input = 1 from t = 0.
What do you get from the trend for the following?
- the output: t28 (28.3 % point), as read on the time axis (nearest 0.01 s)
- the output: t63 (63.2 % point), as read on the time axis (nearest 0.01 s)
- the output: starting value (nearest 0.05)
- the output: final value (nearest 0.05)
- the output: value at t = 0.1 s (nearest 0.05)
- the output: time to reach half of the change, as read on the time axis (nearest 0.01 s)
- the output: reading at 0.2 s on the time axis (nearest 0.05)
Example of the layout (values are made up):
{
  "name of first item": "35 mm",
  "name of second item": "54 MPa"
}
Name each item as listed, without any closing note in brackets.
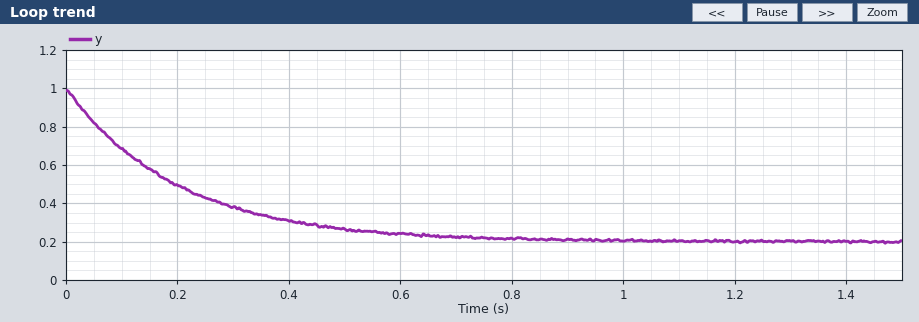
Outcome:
{
  "the output: t28 (28.3 % point), as read on the time axis": "0.07 s",
  "the output: t63 (63.2 % point), as read on the time axis": "0.20 s",
  "the output: starting value": "1.00",
  "the output: final value": "0.20",
  "the output: value at t = 0.1 s": "0.70",
  "the output: time to reach half of the change, as read on the time axis": "0.14 s",
  "the output: reading at 0.2 s on the time axis": "0.50"
}
